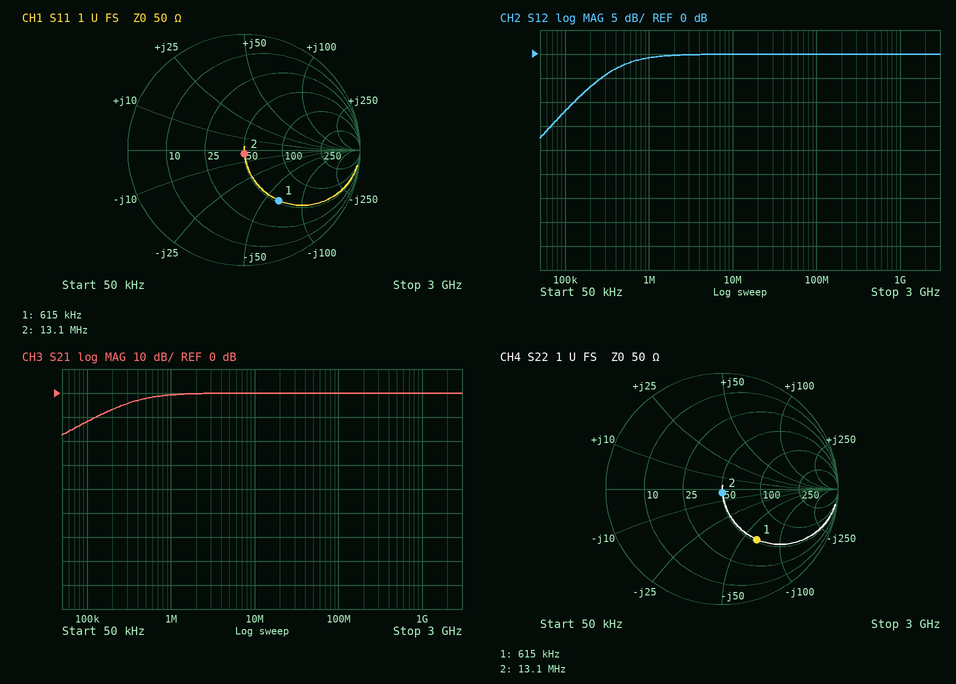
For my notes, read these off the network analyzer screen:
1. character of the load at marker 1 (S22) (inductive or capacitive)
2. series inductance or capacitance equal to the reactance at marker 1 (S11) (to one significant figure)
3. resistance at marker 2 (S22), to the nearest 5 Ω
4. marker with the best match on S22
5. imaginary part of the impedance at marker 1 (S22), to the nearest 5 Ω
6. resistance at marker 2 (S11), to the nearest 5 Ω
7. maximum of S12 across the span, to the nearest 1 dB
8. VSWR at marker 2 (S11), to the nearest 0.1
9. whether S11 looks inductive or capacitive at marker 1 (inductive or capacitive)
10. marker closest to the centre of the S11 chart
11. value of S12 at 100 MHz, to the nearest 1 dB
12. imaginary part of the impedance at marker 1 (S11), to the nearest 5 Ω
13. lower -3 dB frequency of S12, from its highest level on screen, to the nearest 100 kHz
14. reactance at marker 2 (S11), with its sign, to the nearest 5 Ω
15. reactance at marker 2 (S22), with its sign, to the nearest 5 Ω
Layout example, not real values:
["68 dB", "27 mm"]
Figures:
["capacitive", "4 nF", "50 Ω", "marker 2", "-65 Ω", "50 Ω", "0 dB", "1.1", "capacitive", "marker 2", "0 dB", "-65 Ω", "400 kHz", "-5 Ω", "-5 Ω"]
